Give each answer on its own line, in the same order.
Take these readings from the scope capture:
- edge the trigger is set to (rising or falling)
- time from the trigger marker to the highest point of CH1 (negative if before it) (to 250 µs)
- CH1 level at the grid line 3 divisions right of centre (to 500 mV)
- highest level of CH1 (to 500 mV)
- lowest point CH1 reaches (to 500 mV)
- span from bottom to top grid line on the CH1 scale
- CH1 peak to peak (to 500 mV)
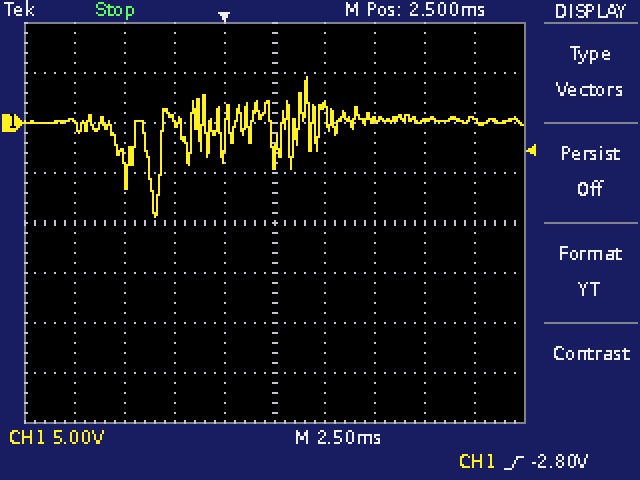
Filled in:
rising
+4.00 ms
0.0 V
4.5 V
-9.5 V
40 V
14.0 V
